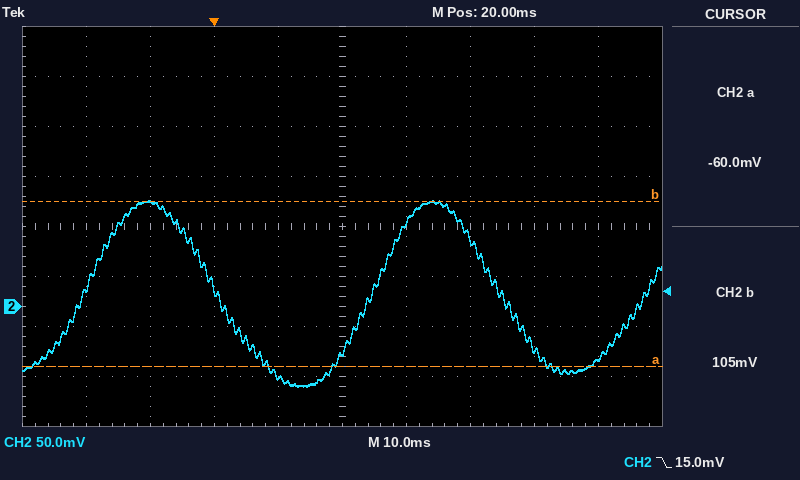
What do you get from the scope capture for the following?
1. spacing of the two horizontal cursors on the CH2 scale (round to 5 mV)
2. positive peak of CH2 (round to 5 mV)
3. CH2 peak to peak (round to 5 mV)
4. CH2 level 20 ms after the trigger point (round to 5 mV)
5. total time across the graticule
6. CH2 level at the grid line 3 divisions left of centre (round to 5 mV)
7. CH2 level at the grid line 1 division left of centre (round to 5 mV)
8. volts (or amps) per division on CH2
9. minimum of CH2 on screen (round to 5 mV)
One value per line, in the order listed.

165 mV
105 mV
185 mV
-45 mV
100 ms
105 mV
-70 mV
50 mV
-80 mV
